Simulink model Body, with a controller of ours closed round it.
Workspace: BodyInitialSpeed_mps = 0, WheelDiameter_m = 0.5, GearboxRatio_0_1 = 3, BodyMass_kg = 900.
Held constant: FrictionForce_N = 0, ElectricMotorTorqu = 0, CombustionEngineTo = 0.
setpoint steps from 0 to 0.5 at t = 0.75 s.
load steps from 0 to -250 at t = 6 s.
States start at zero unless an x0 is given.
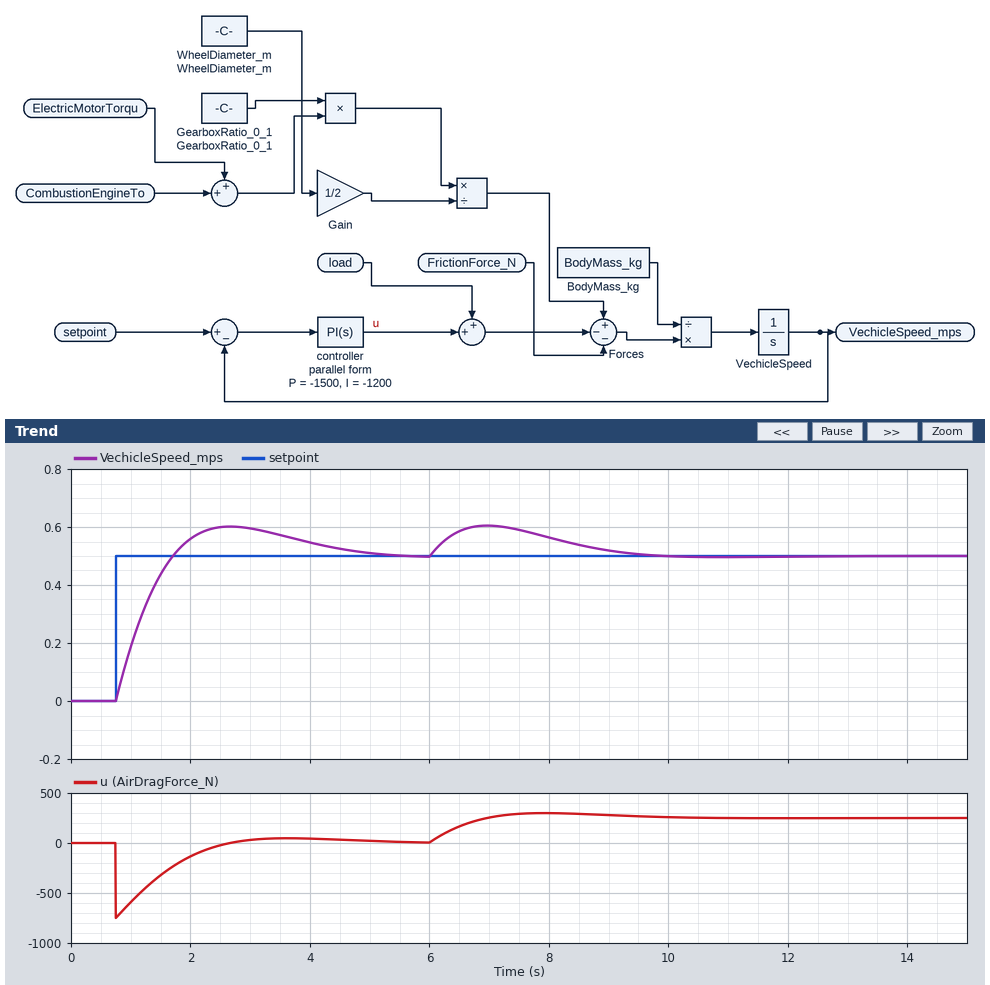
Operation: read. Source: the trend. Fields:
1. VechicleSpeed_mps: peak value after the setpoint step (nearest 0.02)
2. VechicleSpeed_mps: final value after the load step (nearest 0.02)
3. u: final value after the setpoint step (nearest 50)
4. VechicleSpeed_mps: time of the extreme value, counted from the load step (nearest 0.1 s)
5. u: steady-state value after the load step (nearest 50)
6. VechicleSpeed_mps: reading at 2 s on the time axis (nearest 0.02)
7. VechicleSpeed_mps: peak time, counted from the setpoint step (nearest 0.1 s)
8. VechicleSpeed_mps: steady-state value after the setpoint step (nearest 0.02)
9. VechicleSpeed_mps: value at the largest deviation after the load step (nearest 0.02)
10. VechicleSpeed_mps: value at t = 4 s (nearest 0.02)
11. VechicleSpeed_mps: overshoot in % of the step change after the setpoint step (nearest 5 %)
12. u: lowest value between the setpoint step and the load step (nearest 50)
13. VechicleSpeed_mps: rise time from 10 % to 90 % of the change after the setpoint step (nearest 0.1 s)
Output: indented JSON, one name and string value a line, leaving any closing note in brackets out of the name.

{
  "VechicleSpeed_mps: peak value after the setpoint step": "0.60",
  "VechicleSpeed_mps: final value after the load step": "0.50",
  "u: final value after the setpoint step": "0",
  "VechicleSpeed_mps: time of the extreme value, counted from the load step": "1.0 s",
  "u: steady-state value after the load step": "250",
  "VechicleSpeed_mps: reading at 2 s on the time axis": "0.56",
  "VechicleSpeed_mps: peak time, counted from the setpoint step": "1.9 s",
  "VechicleSpeed_mps: steady-state value after the setpoint step": "0.50",
  "VechicleSpeed_mps: value at the largest deviation after the load step": "0.60",
  "VechicleSpeed_mps: value at t = 4 s": "0.54",
  "VechicleSpeed_mps: overshoot in % of the step change after the setpoint step": "20 %",
  "u: lowest value between the setpoint step and the load step": "-750",
  "VechicleSpeed_mps: rise time from 10 % to 90 % of the change after the setpoint step": "0.7 s"
}
